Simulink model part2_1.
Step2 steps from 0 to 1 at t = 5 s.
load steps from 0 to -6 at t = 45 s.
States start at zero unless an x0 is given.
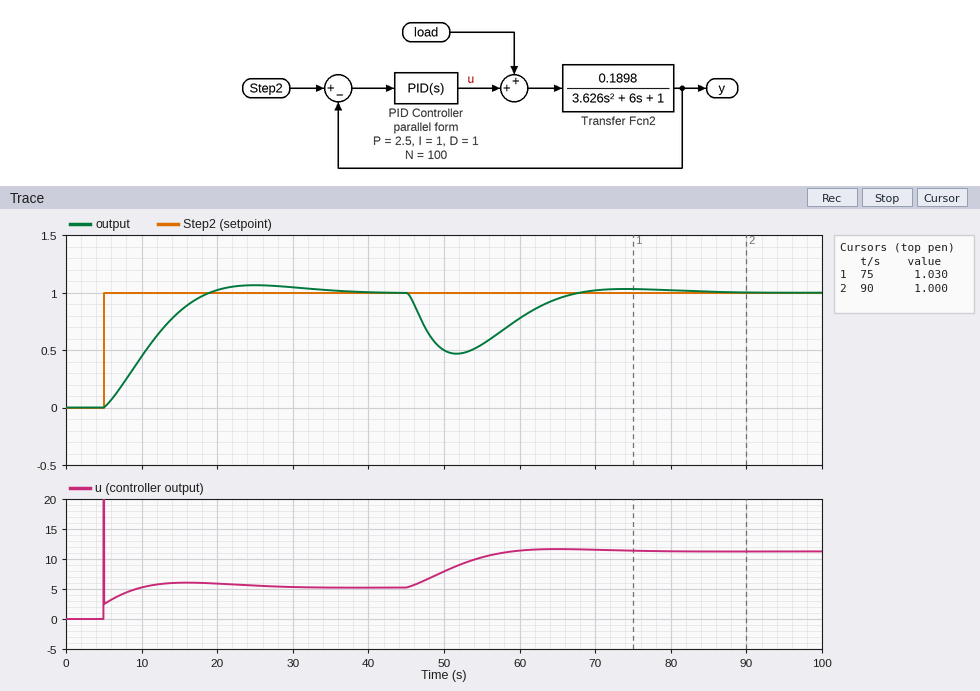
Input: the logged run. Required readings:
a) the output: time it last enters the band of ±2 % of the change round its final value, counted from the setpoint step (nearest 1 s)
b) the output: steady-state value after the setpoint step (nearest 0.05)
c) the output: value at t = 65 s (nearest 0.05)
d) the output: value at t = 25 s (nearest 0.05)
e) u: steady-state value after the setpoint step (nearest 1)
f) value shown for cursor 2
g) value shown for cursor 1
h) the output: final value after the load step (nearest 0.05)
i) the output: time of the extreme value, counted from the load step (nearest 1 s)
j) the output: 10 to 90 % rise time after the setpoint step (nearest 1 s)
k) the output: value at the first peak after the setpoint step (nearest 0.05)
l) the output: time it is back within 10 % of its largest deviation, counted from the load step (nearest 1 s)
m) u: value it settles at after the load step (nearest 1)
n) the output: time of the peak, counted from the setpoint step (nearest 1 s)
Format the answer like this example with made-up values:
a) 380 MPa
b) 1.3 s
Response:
a) 30 s
b) 1.00
c) 0.95
d) 1.05
e) 5
f) 1.000
g) 1.030
h) 1.00
i) 7 s
j) 10 s
k) 1.05
l) 20 s
m) 11
n) 20 s
